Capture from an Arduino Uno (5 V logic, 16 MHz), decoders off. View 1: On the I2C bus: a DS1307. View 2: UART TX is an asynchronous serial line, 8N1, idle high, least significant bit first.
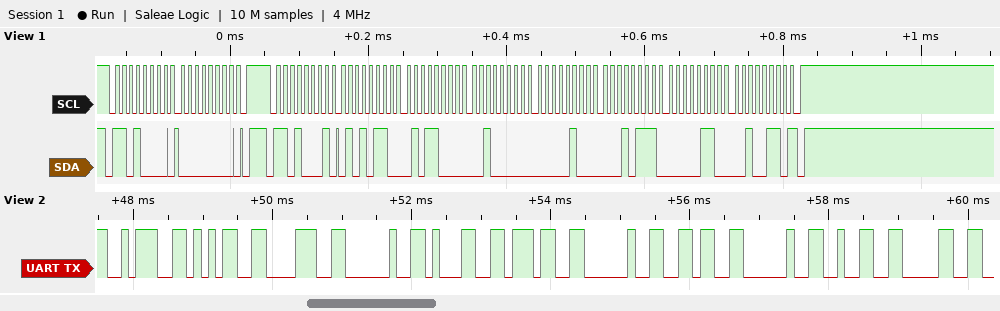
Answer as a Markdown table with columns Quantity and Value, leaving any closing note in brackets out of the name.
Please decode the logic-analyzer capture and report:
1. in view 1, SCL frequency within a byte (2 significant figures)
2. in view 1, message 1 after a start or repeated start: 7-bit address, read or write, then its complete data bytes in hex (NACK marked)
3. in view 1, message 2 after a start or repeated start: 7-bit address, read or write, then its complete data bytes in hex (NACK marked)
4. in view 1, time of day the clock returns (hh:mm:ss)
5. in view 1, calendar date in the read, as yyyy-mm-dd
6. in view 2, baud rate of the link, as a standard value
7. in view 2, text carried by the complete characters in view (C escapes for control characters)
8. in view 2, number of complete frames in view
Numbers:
| Quantity | Value |
|---|---|
| in view 1, SCL frequency within a byte | 100 kHz |
| in view 1, message 1 after a start or repeated start: 7-bit address, read or write, then its complete data bytes in hex | 0x68 write: 00 |
| in view 1, message 2 after a start or repeated start: 7-bit address, read or write, then its complete data bytes in hex | 0x68 read: 56 58 20 04 17 06 26 NACK |
| in view 1, time of day the clock returns | 20:58:56 |
| in view 1, calendar date in the read, as yyyy-mm-dd | 2026-06-17 |
| in view 2, baud rate of the link, as a standard value | 9600 baud |
| in view 2, text carried by the complete characters in view | ":58 17 6 20" |
| in view 2, number of complete frames in view | 11 |
